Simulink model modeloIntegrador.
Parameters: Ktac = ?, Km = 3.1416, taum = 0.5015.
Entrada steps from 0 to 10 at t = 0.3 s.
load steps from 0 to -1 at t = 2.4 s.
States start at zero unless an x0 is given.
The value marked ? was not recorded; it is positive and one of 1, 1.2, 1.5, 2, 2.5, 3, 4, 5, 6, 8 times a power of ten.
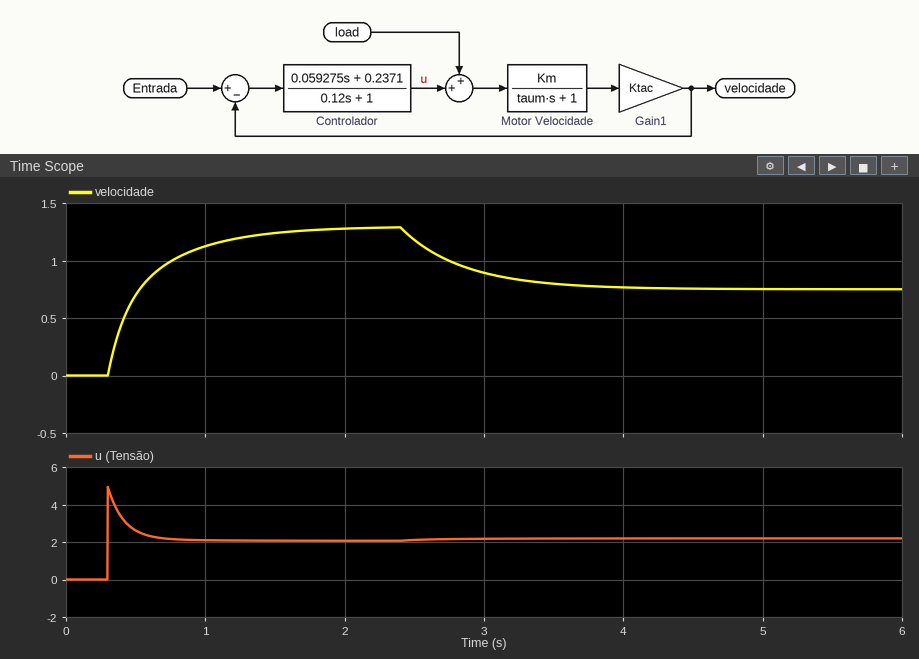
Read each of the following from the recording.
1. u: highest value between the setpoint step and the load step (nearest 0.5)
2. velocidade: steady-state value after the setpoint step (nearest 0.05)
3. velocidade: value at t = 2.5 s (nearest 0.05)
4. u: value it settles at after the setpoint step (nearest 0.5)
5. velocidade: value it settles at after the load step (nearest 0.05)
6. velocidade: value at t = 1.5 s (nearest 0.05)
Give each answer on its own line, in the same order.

5.0
1.30
1.20
2.0
0.75
1.25
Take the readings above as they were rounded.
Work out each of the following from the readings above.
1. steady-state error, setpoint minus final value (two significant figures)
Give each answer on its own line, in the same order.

8.7
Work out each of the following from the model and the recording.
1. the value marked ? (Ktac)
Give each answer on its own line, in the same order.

0.2
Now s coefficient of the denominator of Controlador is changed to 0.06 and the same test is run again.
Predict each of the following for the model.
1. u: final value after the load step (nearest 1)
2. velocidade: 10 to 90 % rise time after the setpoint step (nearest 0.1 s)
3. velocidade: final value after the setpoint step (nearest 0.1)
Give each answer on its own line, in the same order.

2
0.8 s
1.3
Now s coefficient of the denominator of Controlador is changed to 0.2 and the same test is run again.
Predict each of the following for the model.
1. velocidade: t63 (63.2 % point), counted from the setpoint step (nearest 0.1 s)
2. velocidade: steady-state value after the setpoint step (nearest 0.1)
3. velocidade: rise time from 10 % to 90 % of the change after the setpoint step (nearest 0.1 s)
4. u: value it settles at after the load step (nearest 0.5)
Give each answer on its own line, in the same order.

0.4 s
1.3
0.9 s
2.0
